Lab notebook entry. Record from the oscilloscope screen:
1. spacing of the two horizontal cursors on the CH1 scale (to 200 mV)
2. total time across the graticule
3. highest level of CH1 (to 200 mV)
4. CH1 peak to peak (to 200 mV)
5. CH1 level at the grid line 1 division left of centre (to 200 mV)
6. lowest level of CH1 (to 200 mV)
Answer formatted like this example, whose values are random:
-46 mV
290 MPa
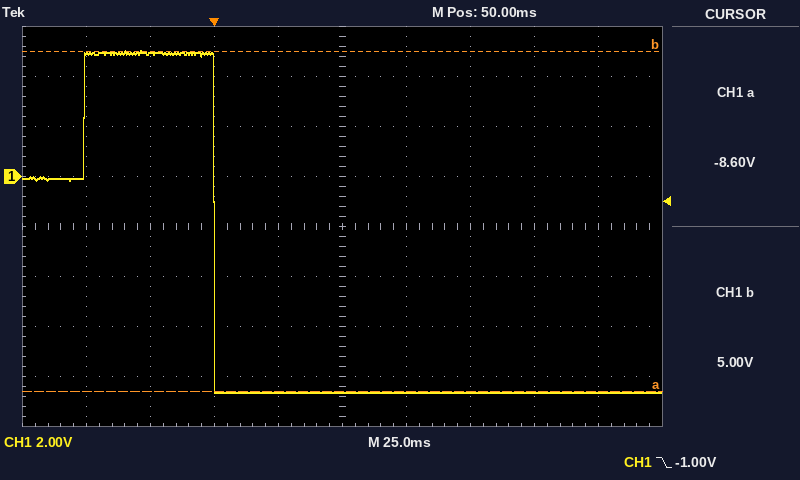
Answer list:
13.6 V
250 ms
5.0 V
13.6 V
-8.6 V
-8.6 V
